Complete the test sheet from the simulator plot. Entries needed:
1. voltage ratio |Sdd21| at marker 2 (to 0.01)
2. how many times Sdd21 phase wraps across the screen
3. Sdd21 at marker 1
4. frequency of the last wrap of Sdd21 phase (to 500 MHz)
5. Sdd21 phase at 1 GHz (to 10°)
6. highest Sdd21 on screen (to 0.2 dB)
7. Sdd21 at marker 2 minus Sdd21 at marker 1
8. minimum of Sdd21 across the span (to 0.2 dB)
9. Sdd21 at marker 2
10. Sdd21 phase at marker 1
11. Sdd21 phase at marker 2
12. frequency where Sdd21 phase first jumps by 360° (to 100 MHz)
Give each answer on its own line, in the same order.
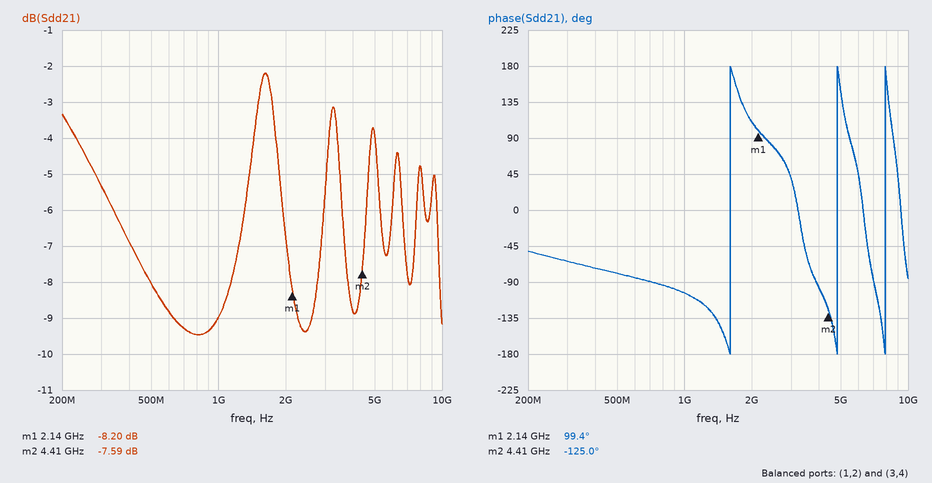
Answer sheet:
0.42
3
-8.20 dB
8.0 GHz
-100°
-2.2 dB
0.61 dB
-9.4 dB
-7.59 dB
99.4°
-125.0°
1.6 GHz
